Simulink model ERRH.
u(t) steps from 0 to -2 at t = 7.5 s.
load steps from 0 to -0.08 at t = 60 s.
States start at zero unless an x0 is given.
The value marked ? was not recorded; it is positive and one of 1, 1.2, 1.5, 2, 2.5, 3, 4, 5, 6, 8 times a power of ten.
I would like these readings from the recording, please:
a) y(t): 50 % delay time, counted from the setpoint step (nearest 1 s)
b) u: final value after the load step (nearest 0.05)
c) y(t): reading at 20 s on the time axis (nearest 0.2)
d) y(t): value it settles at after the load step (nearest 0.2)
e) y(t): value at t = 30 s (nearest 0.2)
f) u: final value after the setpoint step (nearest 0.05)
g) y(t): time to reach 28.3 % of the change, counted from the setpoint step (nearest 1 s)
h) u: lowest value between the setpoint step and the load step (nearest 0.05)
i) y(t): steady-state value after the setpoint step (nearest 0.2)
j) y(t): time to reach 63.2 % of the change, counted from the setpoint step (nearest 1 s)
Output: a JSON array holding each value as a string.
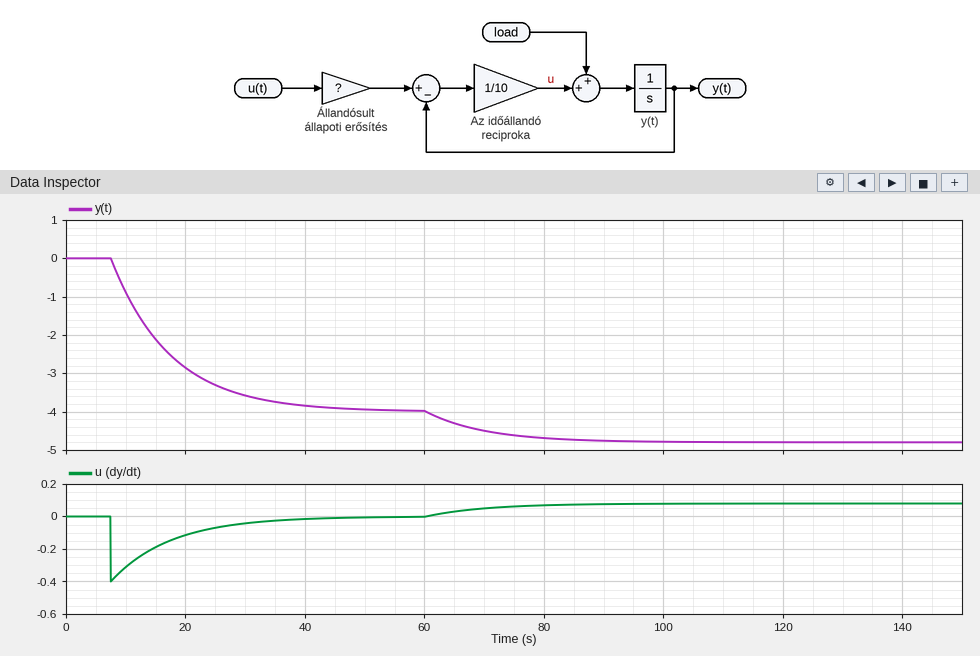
["7 s", "0.10", "-2.8", "-4.8", "-3.6", "0.00", "3 s", "-0.40", "-4.0", "10 s"]
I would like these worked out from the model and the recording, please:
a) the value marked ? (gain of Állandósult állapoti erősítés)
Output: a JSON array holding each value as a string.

["2"]
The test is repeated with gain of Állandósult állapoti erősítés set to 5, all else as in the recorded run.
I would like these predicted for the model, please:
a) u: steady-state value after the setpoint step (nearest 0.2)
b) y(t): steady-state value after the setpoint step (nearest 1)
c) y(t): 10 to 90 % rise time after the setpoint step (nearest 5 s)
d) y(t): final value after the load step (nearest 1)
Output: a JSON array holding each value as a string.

["0.0", "-10", "20 s", "-11"]
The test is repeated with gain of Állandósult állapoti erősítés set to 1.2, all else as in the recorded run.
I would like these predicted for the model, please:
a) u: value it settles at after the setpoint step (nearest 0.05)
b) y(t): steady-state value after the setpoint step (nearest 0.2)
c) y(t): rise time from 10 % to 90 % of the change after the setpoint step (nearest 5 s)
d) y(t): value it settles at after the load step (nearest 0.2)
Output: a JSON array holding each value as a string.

["0.00", "-2.4", "20 s", "-3.2"]
